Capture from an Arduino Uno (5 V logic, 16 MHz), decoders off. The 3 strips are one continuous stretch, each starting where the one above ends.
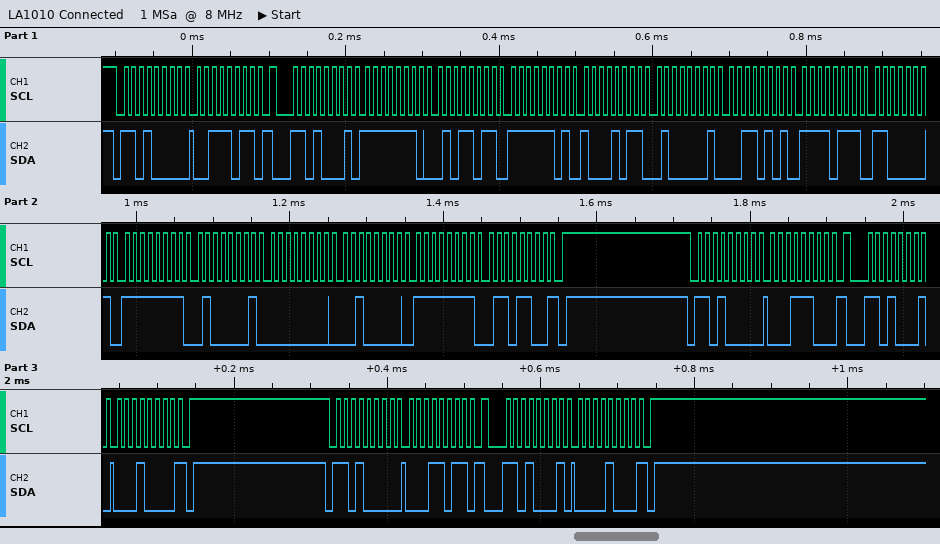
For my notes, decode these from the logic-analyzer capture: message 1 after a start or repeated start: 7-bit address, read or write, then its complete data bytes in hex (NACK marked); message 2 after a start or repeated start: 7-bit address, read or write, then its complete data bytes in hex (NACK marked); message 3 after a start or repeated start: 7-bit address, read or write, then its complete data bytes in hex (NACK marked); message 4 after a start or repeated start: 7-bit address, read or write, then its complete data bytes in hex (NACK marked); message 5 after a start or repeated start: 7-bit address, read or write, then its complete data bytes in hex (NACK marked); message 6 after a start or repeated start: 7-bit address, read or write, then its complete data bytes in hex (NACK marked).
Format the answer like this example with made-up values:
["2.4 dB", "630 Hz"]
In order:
["0x68 write: 3B", "0x68 read: FE 5B FD 8B 41 35 F7 C1 FF 41 00 20 FF 6C NACK", "0x68 write: 1C", "0x68 read: 10 NACK", "0x68 write: 1B", "0x68 read: 08 NACK"]
